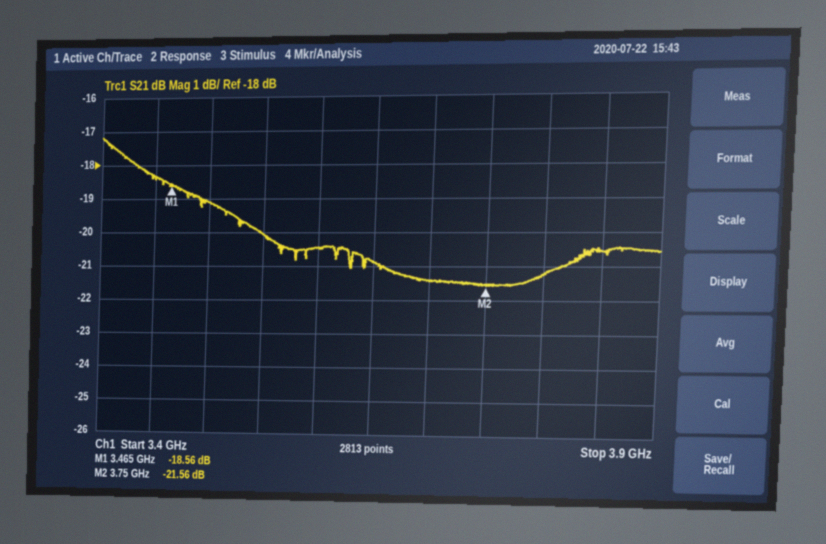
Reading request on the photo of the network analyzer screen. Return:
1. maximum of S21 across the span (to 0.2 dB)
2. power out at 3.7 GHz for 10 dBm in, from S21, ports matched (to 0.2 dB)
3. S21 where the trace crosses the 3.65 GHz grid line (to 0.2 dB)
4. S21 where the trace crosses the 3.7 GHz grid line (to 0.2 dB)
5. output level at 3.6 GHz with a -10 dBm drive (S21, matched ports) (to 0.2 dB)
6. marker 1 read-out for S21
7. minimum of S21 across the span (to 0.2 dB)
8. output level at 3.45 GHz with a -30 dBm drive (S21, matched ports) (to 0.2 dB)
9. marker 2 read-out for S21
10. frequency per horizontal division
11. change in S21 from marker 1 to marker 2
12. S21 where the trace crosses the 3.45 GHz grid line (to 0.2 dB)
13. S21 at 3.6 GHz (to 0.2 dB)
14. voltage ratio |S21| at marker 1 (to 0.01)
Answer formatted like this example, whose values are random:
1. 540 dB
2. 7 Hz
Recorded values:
1. -17.2 dB
2. -11.4 dBm
3. -20.8 dB
4. -21.4 dB
5. -30.4 dBm
6. -18.56 dB
7. -21.6 dB
8. -48.4 dBm
9. -21.56 dB
10. 50 MHz
11. -3.00 dB
12. -18.4 dB
13. -20.4 dB
14. 0.12
